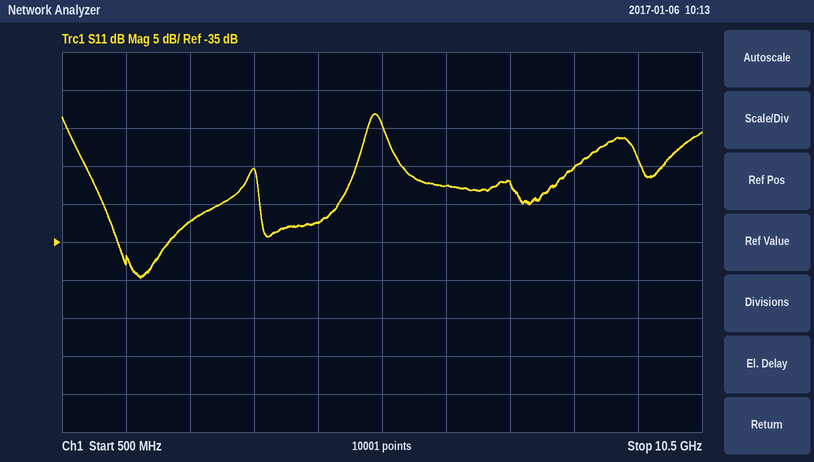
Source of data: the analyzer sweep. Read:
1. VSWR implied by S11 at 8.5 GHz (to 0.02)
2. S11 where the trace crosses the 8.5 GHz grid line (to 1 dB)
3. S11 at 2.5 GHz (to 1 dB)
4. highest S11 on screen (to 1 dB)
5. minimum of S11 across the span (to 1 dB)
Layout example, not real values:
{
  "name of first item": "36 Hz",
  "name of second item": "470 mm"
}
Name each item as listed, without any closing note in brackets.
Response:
{
  "VSWR implied by S11 at 8.5 GHz": "1.12",
  "S11 where the trace crosses the 8.5 GHz grid line": "-25 dB",
  "S11 at 2.5 GHz": "-32 dB",
  "highest S11 on screen": "-18 dB",
  "minimum of S11 across the span": "-40 dB"
}
